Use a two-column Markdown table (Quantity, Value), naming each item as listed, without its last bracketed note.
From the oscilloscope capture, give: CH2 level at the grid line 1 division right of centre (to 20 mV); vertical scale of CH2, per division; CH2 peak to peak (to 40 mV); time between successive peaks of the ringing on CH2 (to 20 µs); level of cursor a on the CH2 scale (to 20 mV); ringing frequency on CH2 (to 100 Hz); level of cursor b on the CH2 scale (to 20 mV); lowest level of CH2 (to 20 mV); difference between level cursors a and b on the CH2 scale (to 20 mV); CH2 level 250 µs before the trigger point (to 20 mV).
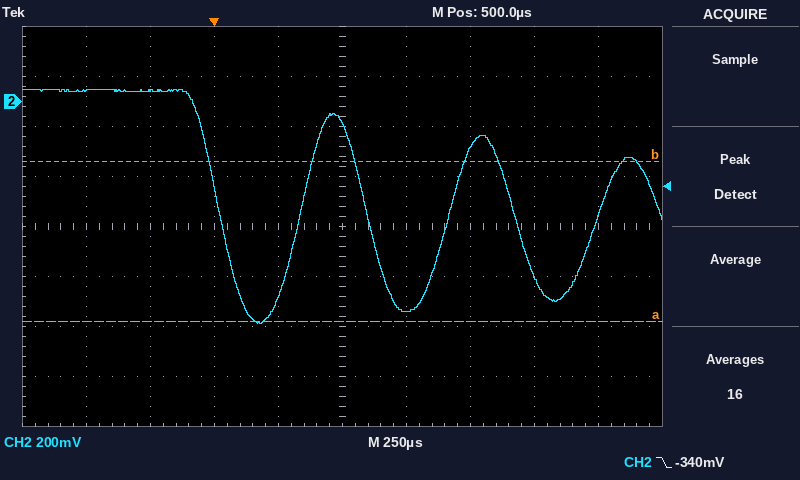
| Quantity | Value |
|---|---|
| CH2 level at the grid line 1 division right of centre | -840 mV |
| vertical scale of CH2, per division | 200 mV |
| CH2 peak to peak | 920 mV |
| time between successive peaks of the ringing on CH2 | 580 µs |
| level of cursor a on the CH2 scale | -880 mV |
| ringing frequency on CH2 | 1.7 kHz |
| level of cursor b on the CH2 scale | -240 mV |
| lowest level of CH2 | -880 mV |
| difference between level cursors a and b on the CH2 scale | 640 mV |
| CH2 level 250 µs before the trigger point | 40 mV |
